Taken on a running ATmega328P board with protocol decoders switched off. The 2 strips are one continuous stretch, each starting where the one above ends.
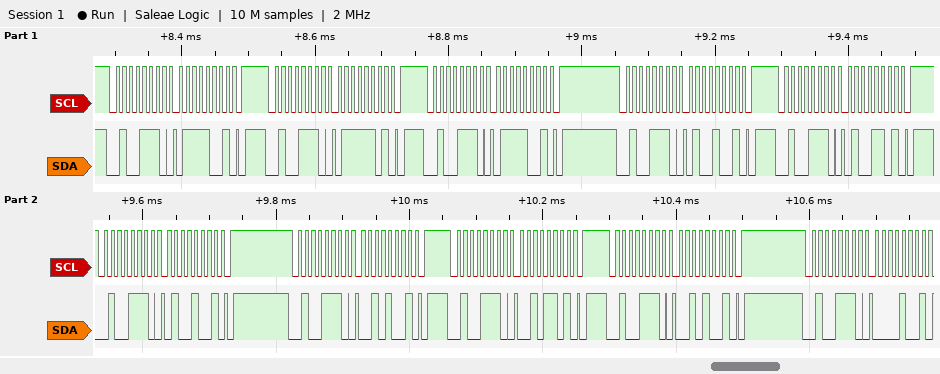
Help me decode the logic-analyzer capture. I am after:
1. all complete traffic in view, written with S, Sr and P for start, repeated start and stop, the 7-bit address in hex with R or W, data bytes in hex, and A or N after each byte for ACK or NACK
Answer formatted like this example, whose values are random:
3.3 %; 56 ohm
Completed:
S 27W A 79 A P S 27W A 7D A P S 27W A 79 A P S 27W A 49 A P S 27W A 4D A P S 27W A 49 A P S 27W A 29 A P S 27W A 2D A P S 27W A 29 A P S 27W A 09 A
